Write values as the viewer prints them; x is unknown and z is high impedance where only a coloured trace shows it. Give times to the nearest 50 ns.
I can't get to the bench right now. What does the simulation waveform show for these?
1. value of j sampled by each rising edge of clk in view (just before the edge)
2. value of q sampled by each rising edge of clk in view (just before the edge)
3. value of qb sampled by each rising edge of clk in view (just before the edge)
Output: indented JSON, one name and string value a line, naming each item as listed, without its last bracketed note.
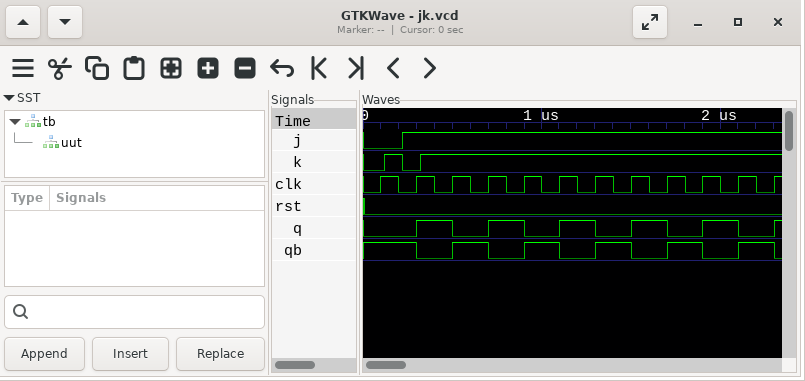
{
  "value of j sampled by each rising edge of clk in view": "0 1 1 1 1 1 1 1 1 1 1 1",
  "value of q sampled by each rising edge of clk in view": "0 0 1 0 1 0 1 0 1 0 1 0",
  "value of qb sampled by each rising edge of clk in view": "1 1 0 1 0 1 0 1 0 1 0 1"
}
